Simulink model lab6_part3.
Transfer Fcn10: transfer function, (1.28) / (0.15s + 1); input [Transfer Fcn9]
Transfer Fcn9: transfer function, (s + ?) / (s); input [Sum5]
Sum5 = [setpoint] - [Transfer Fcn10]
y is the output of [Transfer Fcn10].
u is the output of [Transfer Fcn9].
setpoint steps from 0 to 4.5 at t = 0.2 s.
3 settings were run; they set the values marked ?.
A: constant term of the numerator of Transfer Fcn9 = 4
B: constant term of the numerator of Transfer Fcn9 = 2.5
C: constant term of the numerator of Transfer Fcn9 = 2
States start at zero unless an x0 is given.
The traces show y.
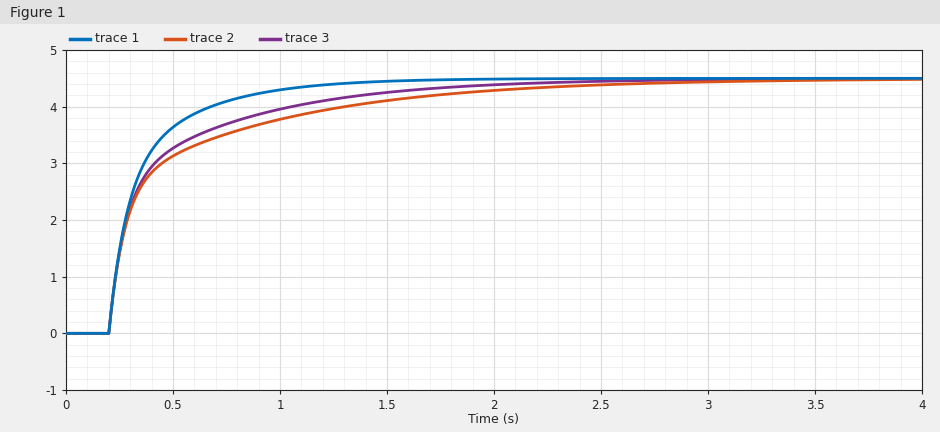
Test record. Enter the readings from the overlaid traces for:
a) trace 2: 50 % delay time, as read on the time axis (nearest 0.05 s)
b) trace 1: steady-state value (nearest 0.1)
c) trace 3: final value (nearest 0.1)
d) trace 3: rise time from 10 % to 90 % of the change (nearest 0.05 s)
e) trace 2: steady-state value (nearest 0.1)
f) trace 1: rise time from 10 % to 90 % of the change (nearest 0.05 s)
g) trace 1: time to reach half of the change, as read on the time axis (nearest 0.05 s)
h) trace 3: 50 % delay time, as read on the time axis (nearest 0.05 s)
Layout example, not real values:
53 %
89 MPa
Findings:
0.30 s
4.5
4.5
0.90 s
4.5
0.50 s
0.30 s
0.30 s
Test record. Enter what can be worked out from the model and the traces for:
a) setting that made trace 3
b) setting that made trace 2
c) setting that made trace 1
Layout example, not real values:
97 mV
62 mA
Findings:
B
C
A
